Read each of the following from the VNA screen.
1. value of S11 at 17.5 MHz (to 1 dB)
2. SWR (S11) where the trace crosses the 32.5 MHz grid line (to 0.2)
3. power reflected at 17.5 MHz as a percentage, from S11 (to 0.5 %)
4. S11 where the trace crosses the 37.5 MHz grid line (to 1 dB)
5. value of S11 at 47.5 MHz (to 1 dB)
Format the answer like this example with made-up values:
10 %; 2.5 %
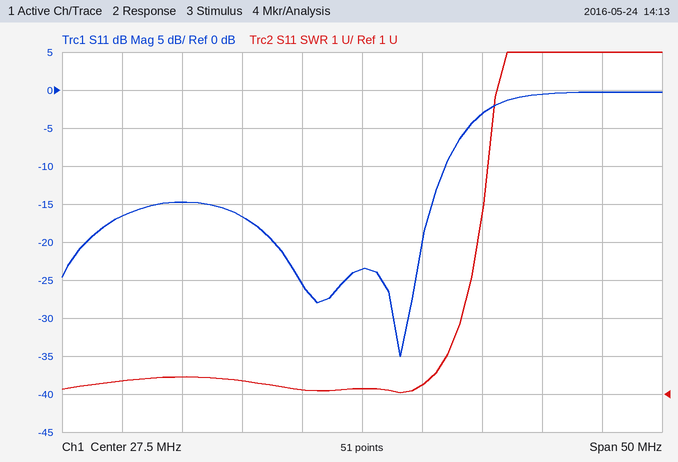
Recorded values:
-17 dB; 1.2; 2.0 %; -3 dB; 0 dB
